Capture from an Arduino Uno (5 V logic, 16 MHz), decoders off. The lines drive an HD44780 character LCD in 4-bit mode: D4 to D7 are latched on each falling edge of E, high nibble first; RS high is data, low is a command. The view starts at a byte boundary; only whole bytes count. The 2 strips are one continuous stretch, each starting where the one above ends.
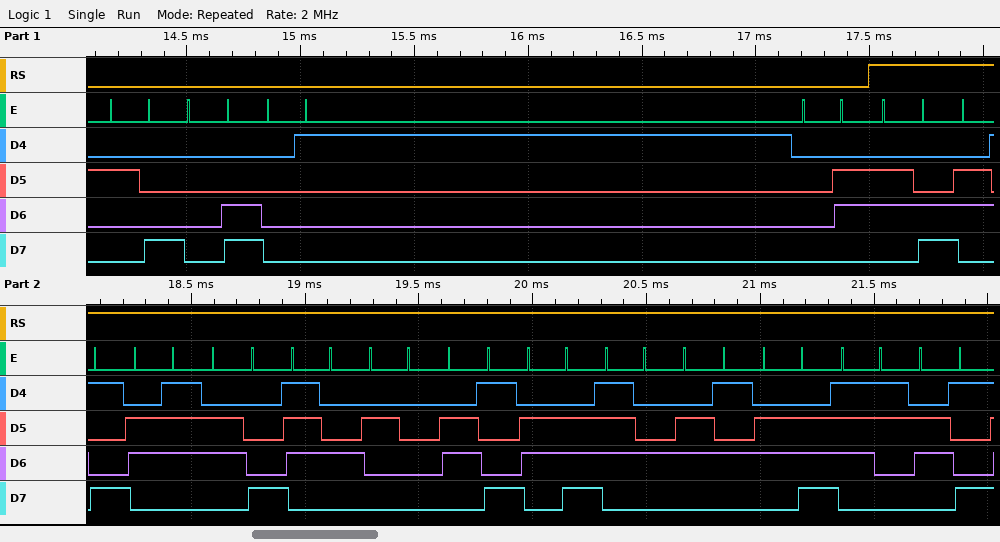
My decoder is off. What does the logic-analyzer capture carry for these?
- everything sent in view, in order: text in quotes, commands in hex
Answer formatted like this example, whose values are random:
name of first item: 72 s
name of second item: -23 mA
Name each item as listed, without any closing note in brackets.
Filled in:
everything sent in view, in order: text in quotes, commands in hex: 0x28 0x0C 0x01 0x06 "light intensi"
